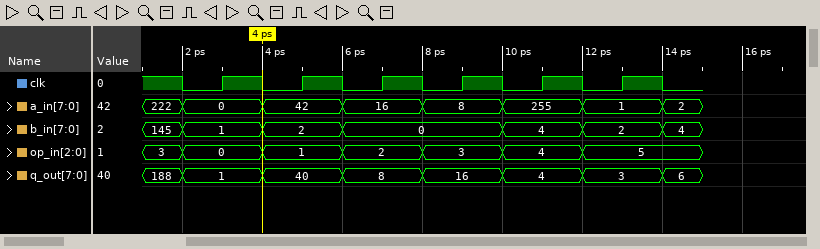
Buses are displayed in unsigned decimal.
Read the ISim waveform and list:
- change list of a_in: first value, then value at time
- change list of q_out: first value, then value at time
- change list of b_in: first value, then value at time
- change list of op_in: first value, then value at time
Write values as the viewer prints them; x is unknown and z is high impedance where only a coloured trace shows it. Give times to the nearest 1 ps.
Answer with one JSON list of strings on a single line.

["222, 0 at 2 ps, 42 at 4 ps, 16 at 6 ps, 8 at 8 ps, 255 at 10 ps, 1 at 12 ps, 2 at 14 ps", "188, 1 at 2 ps, 40 at 4 ps, 8 at 6 ps, 16 at 8 ps, 4 at 10 ps, 3 at 12 ps, 6 at 14 ps", "145, 1 at 2 ps, 2 at 4 ps, 0 at 6 ps, 4 at 10 ps, 2 at 12 ps, 4 at 14 ps", "3, 0 at 2 ps, 1 at 4 ps, 2 at 6 ps, 3 at 8 ps, 4 at 10 ps, 5 at 12 ps"]
